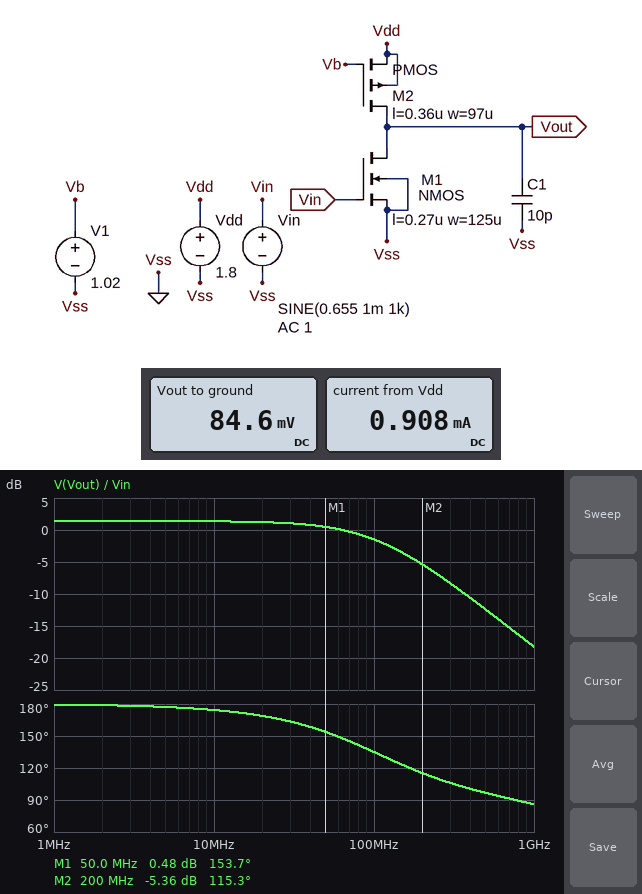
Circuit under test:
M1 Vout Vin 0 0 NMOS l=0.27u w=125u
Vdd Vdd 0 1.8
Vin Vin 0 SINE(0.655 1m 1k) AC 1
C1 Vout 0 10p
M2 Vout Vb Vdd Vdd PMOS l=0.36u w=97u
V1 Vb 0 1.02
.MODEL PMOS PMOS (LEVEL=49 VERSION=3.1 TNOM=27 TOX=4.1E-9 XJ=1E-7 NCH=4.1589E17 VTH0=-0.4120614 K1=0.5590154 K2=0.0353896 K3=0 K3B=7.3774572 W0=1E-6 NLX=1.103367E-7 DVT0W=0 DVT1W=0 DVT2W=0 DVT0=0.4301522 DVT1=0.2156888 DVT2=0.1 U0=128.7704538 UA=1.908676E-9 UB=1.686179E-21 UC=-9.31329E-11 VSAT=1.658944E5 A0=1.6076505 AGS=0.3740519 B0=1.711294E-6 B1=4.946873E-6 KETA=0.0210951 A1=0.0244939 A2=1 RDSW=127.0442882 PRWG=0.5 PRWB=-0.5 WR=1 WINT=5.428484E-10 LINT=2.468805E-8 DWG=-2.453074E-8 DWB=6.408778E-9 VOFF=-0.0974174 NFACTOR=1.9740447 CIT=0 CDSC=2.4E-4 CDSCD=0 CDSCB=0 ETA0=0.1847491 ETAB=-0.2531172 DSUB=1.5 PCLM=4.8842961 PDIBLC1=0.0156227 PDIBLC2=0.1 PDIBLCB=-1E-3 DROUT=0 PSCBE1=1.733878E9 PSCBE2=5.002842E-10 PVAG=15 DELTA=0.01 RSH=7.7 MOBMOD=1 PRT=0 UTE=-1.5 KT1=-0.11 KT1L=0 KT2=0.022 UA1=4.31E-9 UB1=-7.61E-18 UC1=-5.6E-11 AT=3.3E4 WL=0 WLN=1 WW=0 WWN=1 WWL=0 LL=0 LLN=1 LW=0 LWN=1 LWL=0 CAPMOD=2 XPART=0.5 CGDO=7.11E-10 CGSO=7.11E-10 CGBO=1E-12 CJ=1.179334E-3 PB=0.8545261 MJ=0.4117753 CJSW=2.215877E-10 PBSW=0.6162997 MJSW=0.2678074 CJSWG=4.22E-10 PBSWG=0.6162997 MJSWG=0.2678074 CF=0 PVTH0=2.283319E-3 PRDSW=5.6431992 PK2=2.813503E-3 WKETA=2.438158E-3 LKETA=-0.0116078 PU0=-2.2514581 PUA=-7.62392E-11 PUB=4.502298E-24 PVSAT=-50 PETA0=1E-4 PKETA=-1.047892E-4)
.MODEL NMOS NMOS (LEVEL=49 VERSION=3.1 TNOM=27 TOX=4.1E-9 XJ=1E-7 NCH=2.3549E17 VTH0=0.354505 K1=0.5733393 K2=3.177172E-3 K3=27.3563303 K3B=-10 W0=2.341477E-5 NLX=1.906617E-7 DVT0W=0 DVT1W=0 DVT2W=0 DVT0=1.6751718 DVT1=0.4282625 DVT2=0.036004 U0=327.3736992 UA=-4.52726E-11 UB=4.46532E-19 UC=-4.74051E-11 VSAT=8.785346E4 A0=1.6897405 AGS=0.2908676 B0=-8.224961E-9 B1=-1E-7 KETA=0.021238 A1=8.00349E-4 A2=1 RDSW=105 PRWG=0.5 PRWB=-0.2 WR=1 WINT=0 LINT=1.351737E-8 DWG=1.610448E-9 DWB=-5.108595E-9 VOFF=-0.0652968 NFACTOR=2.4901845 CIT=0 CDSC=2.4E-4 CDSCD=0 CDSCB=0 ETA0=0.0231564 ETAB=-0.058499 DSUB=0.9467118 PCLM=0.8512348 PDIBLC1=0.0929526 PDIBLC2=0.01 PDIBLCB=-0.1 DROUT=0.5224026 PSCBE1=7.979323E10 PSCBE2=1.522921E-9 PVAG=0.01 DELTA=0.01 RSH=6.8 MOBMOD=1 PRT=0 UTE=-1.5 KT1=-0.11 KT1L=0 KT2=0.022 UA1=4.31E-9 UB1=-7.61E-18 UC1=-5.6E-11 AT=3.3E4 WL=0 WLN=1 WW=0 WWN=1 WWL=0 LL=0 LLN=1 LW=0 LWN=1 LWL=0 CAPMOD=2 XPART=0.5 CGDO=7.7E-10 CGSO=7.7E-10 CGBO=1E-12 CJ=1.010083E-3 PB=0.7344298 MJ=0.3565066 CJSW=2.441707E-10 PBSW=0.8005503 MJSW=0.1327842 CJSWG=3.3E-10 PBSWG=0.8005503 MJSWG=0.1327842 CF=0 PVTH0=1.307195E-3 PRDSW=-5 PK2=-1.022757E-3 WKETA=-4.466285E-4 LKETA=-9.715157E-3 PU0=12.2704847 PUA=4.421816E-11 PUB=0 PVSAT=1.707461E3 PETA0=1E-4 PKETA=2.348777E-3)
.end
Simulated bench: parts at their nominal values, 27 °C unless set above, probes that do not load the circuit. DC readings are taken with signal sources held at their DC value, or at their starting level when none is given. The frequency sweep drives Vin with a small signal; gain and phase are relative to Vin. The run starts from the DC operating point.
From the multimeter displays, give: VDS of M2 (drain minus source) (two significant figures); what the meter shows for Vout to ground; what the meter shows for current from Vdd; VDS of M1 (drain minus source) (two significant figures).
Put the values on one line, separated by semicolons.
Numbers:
-1.7 V; 84.6 mV; 0.908 mA; 85 mV
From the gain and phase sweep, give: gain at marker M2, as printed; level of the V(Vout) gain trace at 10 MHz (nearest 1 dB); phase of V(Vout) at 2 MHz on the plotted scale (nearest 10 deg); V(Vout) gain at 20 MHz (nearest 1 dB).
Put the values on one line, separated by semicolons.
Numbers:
-5.36 dB; 1 dB; 180 deg; 1 dB
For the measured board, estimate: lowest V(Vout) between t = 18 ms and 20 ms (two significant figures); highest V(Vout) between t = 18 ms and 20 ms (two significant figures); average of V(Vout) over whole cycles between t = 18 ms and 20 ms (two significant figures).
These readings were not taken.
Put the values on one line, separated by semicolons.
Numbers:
83 mV; 86 mV; 85 mV
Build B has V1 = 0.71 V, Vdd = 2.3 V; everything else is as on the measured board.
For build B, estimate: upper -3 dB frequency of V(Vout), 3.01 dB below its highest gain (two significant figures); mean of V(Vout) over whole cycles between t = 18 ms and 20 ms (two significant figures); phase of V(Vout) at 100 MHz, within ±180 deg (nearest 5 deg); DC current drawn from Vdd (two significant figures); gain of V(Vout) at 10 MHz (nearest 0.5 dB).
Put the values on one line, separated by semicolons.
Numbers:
200 MHz; 2.2 V; 155 deg; 1.7 mA; 2.5 dB
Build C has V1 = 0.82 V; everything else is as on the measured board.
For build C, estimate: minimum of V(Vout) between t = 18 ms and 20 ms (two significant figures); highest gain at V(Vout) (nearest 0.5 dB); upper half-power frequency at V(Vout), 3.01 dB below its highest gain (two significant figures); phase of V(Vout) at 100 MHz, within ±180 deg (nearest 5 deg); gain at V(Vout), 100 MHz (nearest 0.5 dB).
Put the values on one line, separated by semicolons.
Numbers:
1.5 V; 12.5 dB; 60 MHz; 120 deg; 7.0 dB
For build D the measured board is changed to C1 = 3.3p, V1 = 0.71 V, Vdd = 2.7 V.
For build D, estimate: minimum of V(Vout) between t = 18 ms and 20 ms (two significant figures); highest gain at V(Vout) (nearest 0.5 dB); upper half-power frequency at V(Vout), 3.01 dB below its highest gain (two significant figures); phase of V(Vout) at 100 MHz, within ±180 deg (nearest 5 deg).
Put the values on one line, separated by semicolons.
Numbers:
2.6 V; 1.0 dB; 690 MHz; 170 deg
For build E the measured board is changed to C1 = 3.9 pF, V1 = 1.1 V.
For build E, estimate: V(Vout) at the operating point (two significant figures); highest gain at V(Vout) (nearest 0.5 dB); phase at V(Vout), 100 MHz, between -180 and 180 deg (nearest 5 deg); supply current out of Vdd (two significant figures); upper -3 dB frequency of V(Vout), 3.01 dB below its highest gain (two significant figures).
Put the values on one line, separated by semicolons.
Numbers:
41 mV; -9.0 dB; 165 deg; 530 µA; 420 MHz
